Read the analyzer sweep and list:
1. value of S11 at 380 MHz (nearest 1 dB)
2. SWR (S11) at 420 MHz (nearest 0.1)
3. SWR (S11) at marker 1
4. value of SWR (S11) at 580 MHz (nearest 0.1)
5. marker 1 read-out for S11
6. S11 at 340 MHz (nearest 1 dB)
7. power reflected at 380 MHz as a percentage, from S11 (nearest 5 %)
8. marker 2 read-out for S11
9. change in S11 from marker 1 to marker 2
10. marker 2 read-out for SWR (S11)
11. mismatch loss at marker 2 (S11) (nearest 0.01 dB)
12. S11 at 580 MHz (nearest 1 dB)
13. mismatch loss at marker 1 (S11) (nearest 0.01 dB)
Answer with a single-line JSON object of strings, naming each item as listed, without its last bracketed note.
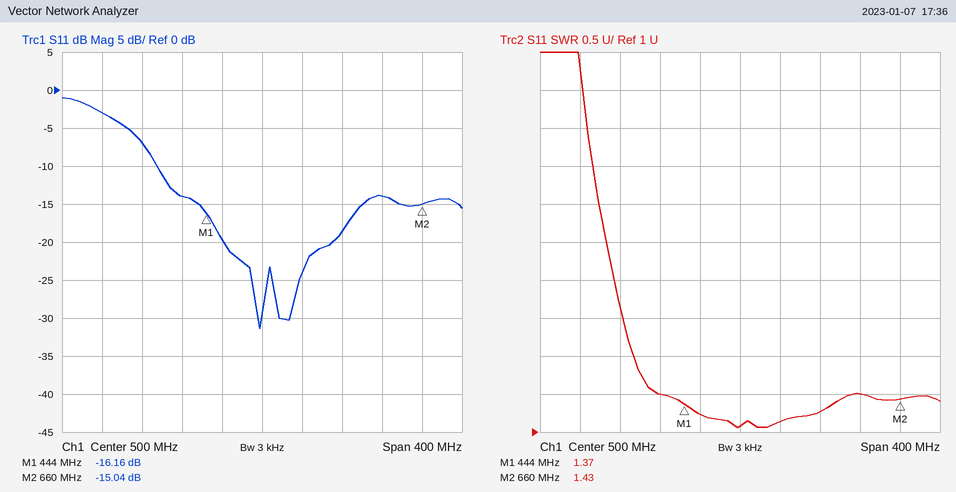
{"value of S11 at 380 MHz": "-7 dB", "SWR (S11) at 420 MHz": "1.5", "SWR (S11) at marker 1": "1.37", "value of SWR (S11) at 580 MHz": "1.3", "marker 1 read-out for S11": "-16.16 dB", "S11 at 340 MHz": "-3 dB", "power reflected at 380 MHz as a percentage, from S11": "20 %", "marker 2 read-out for S11": "-15.04 dB", "change in S11 from marker 1 to marker 2": "1.12 dB", "marker 2 read-out for SWR": "1.43", "mismatch loss at marker 2 (S11)": "0.14 dB", "S11 at 580 MHz": "-19 dB", "mismatch loss at marker 1 (S11)": "0.11 dB"}
